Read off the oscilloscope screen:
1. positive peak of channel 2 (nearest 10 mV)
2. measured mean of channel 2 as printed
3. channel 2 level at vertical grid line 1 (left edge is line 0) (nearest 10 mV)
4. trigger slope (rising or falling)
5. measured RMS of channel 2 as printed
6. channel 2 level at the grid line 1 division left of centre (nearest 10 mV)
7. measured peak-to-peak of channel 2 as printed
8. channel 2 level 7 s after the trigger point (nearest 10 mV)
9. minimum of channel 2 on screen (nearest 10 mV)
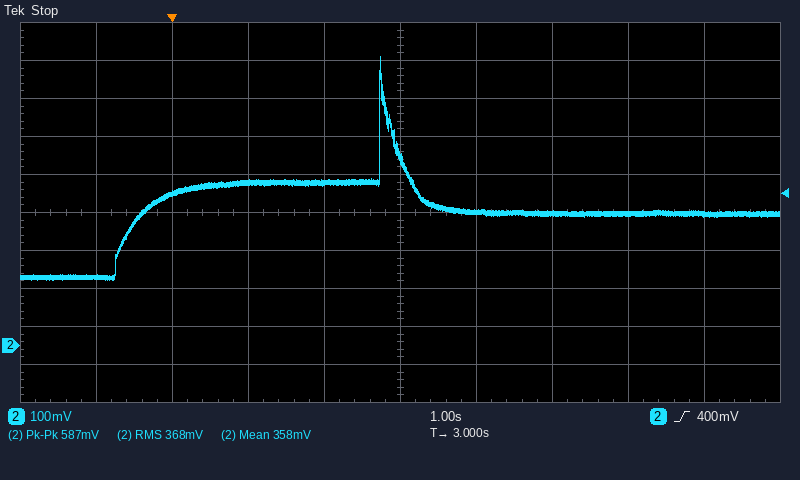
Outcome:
760 mV
358 mV
180 mV
rising
368 mV
430 mV
587 mV
350 mV
170 mV
